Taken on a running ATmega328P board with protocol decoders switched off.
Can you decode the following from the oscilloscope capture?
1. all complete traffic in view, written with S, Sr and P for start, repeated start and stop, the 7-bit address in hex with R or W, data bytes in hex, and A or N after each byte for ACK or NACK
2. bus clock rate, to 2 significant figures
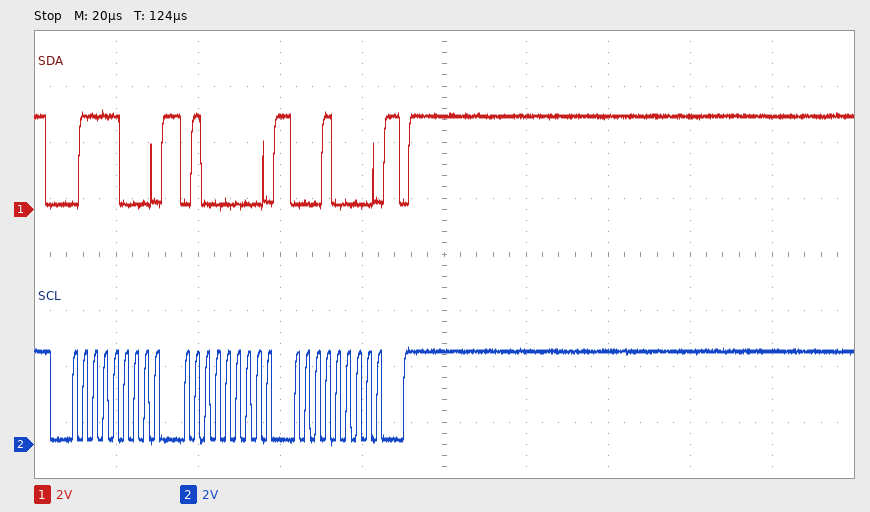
S 3CW A 40 A 10 A P
400 kHz
